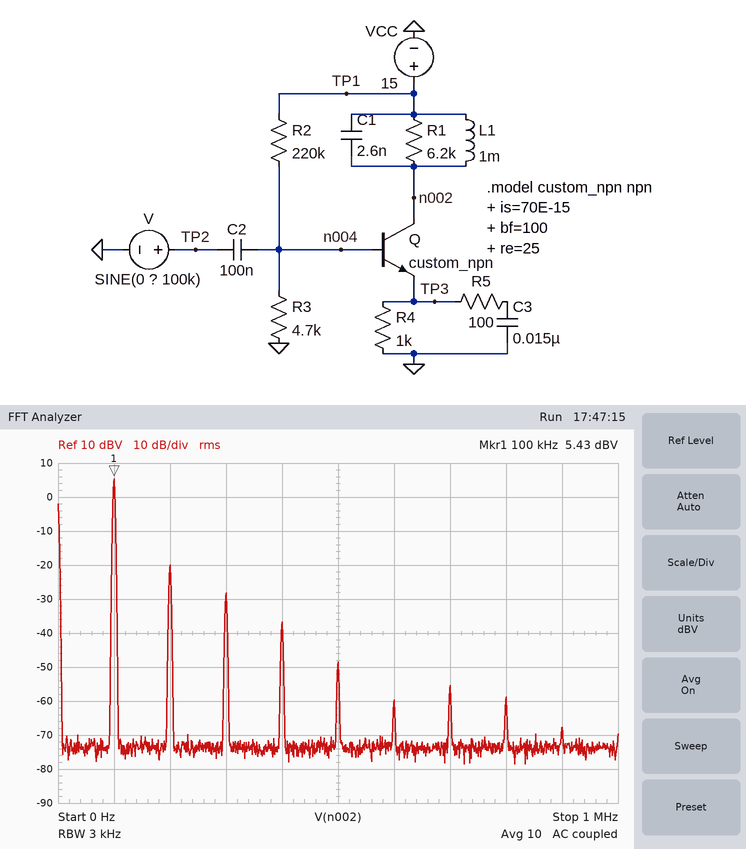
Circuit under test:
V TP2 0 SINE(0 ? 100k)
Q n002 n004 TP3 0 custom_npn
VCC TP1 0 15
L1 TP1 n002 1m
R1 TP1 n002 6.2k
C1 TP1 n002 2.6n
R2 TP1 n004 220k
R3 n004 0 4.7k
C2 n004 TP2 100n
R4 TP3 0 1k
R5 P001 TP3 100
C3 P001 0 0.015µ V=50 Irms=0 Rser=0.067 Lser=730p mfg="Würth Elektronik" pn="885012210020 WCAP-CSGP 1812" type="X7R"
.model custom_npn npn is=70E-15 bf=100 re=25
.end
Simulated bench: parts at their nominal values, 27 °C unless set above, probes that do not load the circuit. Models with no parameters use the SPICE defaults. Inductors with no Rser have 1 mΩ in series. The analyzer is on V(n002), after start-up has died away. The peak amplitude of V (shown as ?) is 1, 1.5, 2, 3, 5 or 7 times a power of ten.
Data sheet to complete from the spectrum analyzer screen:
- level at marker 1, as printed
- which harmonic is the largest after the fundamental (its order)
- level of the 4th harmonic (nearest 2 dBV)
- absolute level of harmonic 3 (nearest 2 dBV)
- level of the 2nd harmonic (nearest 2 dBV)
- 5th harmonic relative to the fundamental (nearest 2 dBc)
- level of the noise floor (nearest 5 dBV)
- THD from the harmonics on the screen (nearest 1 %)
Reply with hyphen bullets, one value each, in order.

- 5.43 dBV
- 2
- -36 dBV
- -28 dBV
- -20 dBV
- -54 dBc
- -75 dBV
- 6 %
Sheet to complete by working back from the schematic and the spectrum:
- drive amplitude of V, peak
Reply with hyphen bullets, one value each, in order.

- 700 mV
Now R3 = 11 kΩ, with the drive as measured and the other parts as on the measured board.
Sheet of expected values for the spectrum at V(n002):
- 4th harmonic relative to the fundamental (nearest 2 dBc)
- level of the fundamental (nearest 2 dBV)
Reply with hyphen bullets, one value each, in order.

- -52 dBc
- 12 dBV
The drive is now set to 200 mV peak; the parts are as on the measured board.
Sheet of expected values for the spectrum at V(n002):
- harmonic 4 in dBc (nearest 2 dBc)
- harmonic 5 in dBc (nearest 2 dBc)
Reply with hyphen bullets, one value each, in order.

- -40 dBc
- -48 dBc
